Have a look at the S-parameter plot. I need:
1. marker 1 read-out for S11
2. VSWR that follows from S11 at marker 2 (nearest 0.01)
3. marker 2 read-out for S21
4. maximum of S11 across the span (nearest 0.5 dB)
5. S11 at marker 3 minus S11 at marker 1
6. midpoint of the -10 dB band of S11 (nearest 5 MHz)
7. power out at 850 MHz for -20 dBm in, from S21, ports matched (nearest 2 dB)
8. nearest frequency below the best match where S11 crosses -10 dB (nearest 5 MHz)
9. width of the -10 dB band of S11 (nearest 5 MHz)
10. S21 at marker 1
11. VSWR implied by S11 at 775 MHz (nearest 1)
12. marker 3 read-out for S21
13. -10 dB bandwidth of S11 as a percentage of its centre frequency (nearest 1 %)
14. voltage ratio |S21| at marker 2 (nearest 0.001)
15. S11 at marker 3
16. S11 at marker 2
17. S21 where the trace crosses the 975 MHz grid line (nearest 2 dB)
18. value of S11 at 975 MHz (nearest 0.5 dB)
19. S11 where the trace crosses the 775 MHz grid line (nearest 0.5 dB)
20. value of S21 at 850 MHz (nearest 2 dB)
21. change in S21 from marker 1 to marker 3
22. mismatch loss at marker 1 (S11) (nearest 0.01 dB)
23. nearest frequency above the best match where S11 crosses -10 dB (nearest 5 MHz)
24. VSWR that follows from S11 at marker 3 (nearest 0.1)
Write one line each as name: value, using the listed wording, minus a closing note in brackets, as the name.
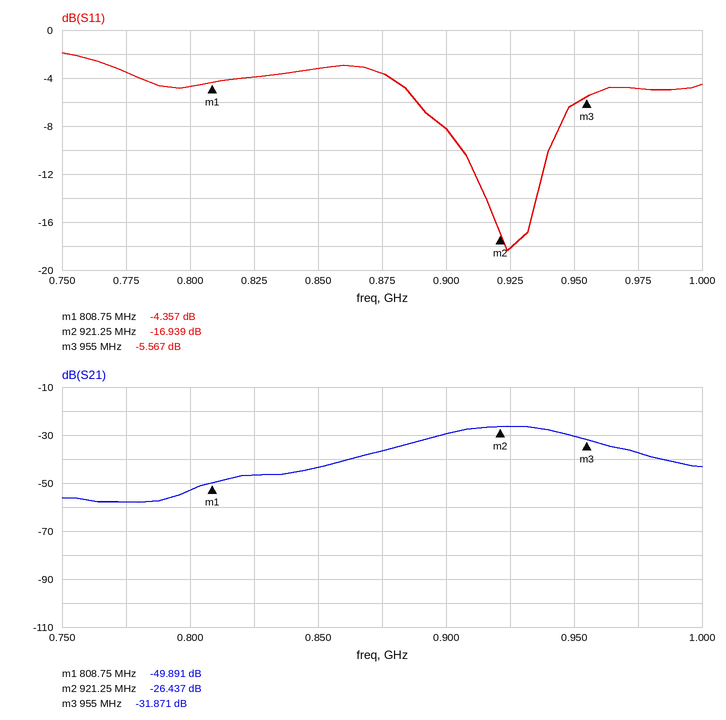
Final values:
marker 1 read-out for S11: -4.357 dB
VSWR that follows from S11 at marker 2: 1.33
marker 2 read-out for S21: -26.437 dB
maximum of S11 across the span: -2.0 dB
S11 at marker 3 minus S11 at marker 1: -1.210 dB
midpoint of the -10 dB band of S11: 925 MHz
power out at 850 MHz for -20 dBm in, from S21, ports matched: -64 dBm
nearest frequency below the best match where S11 crosses -10 dB: 905 MHz
width of the -10 dB band of S11: 35 MHz
S21 at marker 1: -49.891 dB
VSWR implied by S11 at 775 MHz: 5
marker 3 read-out for S21: -31.871 dB
-10 dB bandwidth of S11 as a percentage of its centre frequency: 4 %
voltage ratio |S21| at marker 2: 0.048
S11 at marker 3: -5.567 dB
S11 at marker 2: -16.939 dB
S21 where the trace crosses the 975 MHz grid line: -38 dB
value of S11 at 975 MHz: -5.0 dB
S11 where the trace crosses the 775 MHz grid line: -3.5 dB
value of S21 at 850 MHz: -44 dB
change in S21 from marker 1 to marker 3: 18.020 dB
mismatch loss at marker 1 (S11): 1.98 dB
nearest frequency above the best match where S11 crosses -10 dB: 940 MHz
VSWR that follows from S11 at marker 3: 3.2
